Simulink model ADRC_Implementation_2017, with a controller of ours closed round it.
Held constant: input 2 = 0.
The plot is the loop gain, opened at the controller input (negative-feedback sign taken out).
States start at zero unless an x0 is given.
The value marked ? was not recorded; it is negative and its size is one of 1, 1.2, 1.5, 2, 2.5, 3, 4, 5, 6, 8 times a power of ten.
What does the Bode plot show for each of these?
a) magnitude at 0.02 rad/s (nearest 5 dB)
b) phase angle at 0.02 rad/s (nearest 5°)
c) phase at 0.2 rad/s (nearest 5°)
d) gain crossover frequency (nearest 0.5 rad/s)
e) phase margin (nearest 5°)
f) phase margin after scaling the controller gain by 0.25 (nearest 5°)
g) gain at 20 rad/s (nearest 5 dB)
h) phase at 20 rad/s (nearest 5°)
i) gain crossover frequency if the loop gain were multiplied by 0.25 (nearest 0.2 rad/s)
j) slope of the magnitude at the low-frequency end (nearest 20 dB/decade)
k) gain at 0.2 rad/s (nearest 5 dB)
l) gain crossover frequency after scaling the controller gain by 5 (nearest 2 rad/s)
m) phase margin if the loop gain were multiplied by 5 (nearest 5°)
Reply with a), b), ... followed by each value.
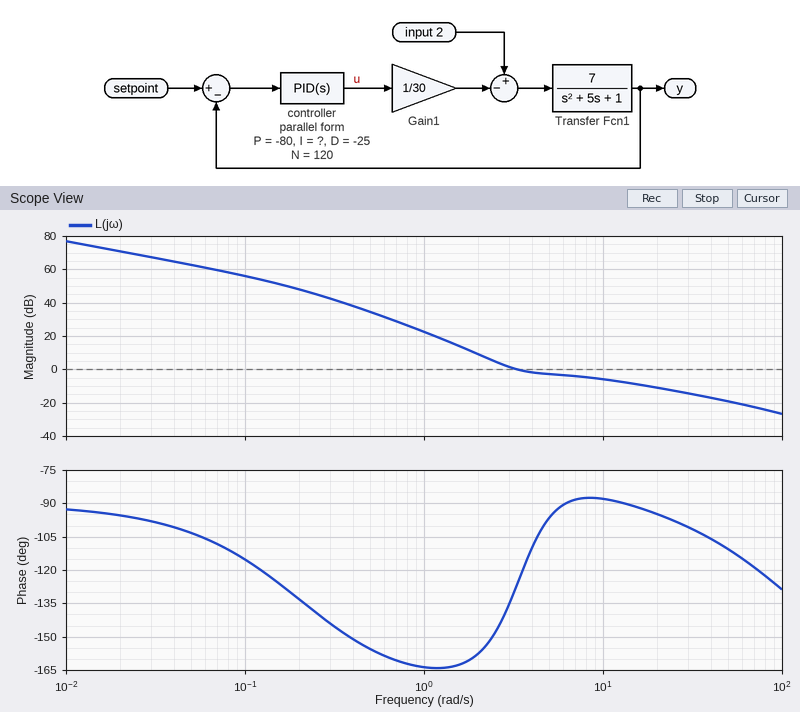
a) 70 dB
b) -95°
c) -135°
d) 3.5 rad/s
e) 55°
f) 20°
g) -10 dB
h) -95°
i) 1.8 rad/s
j) -20 dB/decade
k) 50 dB
l) 28 rad/s
m) 80°
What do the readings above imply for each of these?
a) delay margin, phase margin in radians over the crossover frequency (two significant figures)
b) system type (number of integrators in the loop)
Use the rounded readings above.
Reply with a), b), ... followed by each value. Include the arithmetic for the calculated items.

a) 55 × π / 180 / 3.5 = 0.27 s
b) 1
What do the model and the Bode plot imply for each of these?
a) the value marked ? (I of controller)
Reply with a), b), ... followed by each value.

a) -300
